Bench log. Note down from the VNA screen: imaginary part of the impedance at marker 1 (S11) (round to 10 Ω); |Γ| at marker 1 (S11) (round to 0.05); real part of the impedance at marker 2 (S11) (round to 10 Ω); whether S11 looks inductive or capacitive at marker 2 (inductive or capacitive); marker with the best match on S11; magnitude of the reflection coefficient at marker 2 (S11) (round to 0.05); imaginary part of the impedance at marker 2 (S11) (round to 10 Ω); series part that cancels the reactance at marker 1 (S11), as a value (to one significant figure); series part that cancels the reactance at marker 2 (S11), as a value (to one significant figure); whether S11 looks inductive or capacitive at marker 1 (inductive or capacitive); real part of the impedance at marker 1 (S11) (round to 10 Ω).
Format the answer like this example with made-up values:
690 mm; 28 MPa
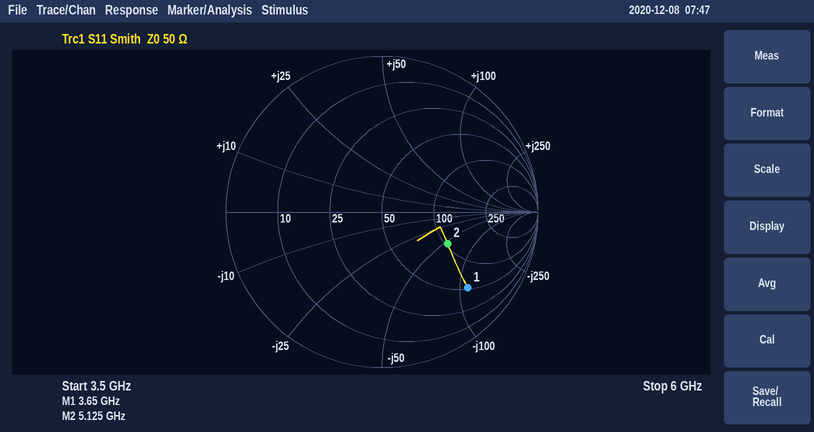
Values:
-110 Ω; 0.75; 100 Ω; capacitive; marker 2; 0.45; -50 Ω; 5 nH; 2 nH; capacitive; 50 Ω
